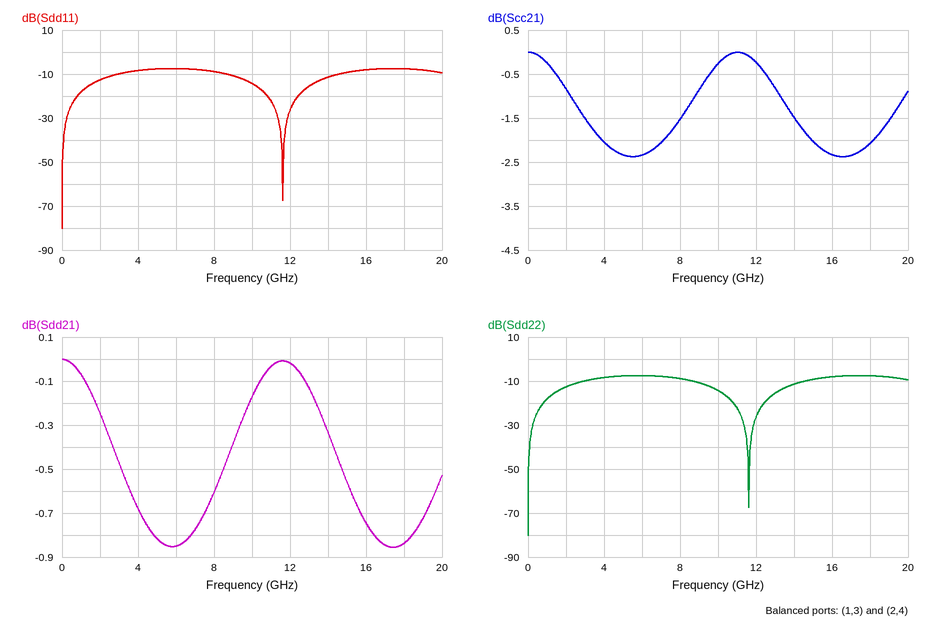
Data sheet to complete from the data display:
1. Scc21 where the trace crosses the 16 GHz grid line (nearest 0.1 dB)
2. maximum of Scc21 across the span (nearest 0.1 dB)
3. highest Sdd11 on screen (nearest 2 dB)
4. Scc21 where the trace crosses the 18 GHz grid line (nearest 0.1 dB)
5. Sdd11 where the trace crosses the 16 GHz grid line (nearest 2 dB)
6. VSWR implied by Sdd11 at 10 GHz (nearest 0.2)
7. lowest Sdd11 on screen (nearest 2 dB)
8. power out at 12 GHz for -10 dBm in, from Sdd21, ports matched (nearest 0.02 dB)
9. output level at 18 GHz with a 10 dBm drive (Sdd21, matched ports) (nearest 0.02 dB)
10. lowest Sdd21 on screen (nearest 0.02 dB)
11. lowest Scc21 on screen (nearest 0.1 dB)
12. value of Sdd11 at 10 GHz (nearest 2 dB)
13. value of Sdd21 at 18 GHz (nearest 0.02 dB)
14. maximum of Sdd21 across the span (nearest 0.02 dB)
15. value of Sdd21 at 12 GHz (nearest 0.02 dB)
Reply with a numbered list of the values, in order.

1. -2.3 dB
2. 0.0 dB
3. -8 dB
4. -2.1 dB
5. -8 dB
6. 1.4
7. -80 dB
8. -10.02 dBm
9. 9.16 dBm
10. -0.86 dB
11. -2.4 dB
12. -14 dB
13. -0.84 dB
14. 0.00 dB
15. -0.02 dB
